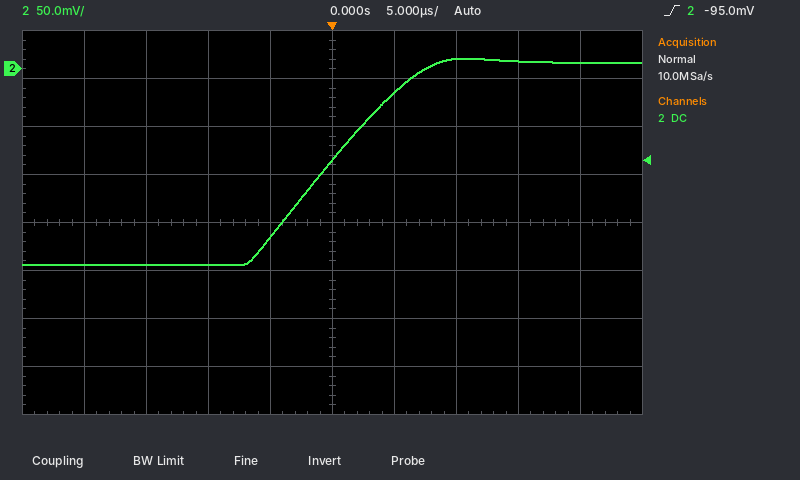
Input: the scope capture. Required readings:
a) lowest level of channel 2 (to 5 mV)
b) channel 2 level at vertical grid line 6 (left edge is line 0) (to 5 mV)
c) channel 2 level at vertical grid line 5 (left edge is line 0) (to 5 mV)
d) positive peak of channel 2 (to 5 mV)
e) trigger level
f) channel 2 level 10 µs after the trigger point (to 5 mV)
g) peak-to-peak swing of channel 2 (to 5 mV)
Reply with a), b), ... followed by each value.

a) -205 mV
b) -25 mV
c) -95 mV
d) 10 mV
e) -95.0 mV
f) 10 mV
g) 215 mV
